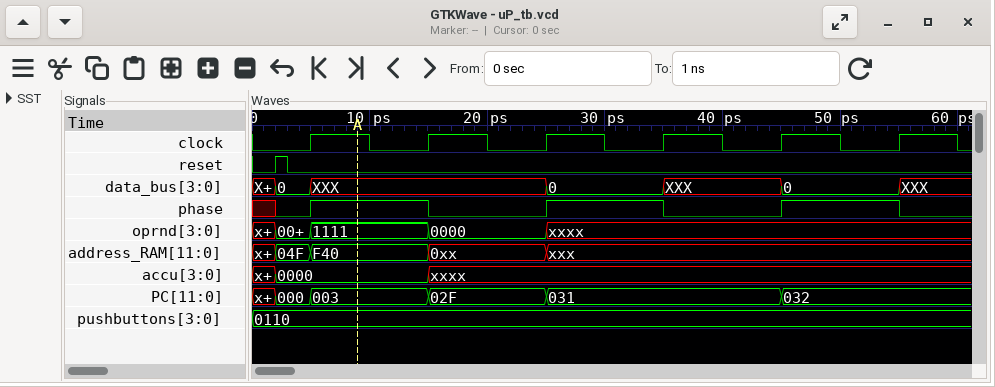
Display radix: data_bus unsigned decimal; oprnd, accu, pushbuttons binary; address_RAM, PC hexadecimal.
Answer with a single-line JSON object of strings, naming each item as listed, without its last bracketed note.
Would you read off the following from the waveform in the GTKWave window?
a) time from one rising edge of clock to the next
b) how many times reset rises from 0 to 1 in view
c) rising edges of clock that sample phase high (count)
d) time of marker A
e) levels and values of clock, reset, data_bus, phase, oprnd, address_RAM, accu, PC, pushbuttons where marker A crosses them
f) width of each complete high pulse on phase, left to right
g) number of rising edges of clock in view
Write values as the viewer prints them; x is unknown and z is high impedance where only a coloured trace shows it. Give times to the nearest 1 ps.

{"time from one rising edge of clock to the next": "10 ps", "how many times reset rises from 0 to 1 in view": "1", "rising edges of clock that sample phase high": "3", "time of marker A": "9 ps", "levels and values of clock, reset, data_bus, phase, oprnd, address_RAM, accu, PC, pushbuttons where marker A crosses them": "clock=1, reset=0, data_bus=XXX, phase=1, oprnd=1111, address_RAM=F40, accu=0000, PC=003, pushbuttons=0110", "width of each complete high pulse on phase, left to right": "10 ps, 10 ps, 10 ps", "number of rising edges of clock in view": "6"}
